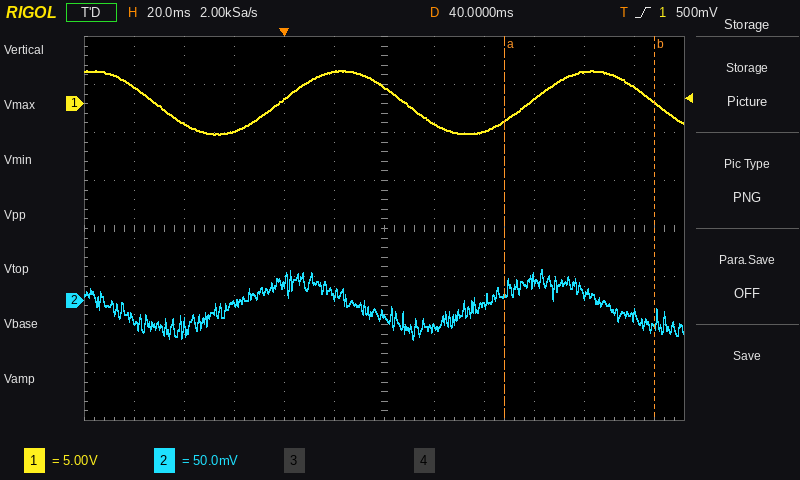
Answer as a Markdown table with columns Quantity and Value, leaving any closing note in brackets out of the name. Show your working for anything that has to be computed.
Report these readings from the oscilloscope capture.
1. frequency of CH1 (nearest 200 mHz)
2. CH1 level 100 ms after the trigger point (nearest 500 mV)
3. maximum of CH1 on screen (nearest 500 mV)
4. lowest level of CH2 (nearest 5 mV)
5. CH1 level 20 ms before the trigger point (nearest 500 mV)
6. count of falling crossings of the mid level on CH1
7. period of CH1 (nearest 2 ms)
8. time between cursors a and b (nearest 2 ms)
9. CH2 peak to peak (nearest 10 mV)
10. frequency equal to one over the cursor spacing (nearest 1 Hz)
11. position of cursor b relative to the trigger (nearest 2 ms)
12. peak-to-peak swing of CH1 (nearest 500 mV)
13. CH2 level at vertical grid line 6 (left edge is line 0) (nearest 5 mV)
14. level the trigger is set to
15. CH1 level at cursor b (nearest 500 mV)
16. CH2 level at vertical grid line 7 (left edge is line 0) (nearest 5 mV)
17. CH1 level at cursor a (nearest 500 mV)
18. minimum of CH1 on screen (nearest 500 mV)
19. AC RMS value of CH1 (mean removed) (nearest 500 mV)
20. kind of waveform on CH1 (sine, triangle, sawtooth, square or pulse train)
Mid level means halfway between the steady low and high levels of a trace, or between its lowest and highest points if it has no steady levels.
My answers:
| Quantity | Value |
|---|---|
| frequency of CH1 | 1 / 100 ms ≈ 10.0 Hz |
| CH1 level 100 ms after the trigger point | 500 mV |
| maximum of CH1 on screen | 3.5 V |
| lowest level of CH2 | -40 mV |
| CH1 level 20 ms before the trigger point | -3.0 V |
| count of falling crossings of the mid level on CH1 | 3 |
| period of CH1 | 100 ms |
| time between cursors a and b | 60 ms |
| CH2 peak to peak | 70 mV |
| frequency equal to one over the cursor spacing | 1 / 60 ms ≈ 17 Hz |
| position of cursor b relative to the trigger | +148 ms |
| peak-to-peak swing of CH1 | 3.5 V − (-3.0 V) = 6.5 V |
| CH2 level at vertical grid line 6 (left edge is line 0) | -15 mV |
| level the trigger is set to | 500 mV |
| CH1 level at cursor b | 0.0 V |
| CH2 level at vertical grid line 7 (left edge is line 0) | -30 mV |
| CH1 level at cursor a | -2.0 V |
| minimum of CH1 on screen | -3.0 V |
| AC RMS value of CH1 (mean removed) | 6.5 V / (2√2) ≈ 2.30 V, so 2.5 V to the nearest 500 mV |
| kind of waveform on CH1 | sine |
